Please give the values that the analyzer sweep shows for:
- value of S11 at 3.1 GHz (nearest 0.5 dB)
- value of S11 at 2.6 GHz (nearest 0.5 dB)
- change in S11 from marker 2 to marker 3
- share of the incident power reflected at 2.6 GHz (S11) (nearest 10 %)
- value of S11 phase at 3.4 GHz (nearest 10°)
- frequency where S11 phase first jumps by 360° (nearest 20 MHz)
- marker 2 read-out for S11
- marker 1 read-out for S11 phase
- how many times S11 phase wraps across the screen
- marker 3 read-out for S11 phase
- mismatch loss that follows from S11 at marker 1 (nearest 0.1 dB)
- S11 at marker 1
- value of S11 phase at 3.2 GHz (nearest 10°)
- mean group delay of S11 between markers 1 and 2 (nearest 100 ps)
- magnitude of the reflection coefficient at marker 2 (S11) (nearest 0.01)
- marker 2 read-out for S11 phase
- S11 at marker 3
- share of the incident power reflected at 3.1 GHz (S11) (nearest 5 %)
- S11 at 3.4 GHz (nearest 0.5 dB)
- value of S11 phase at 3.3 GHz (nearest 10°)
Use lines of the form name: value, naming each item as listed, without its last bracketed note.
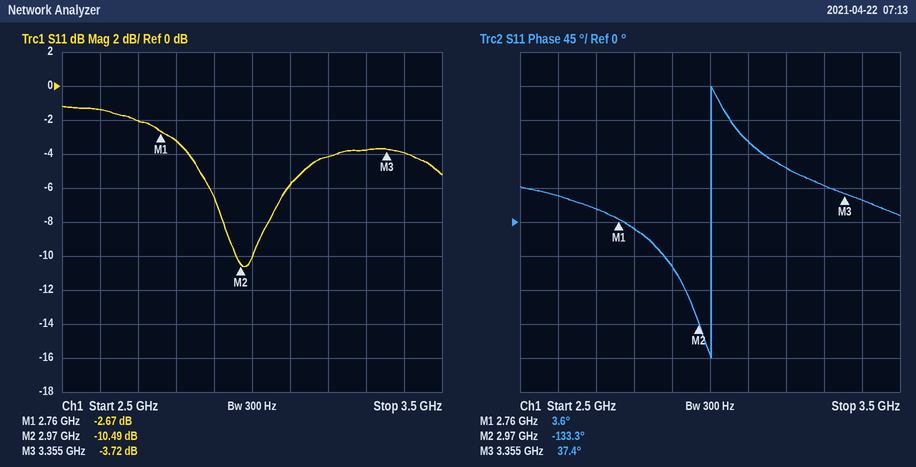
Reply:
value of S11 at 3.1 GHz: -6.0 dB
value of S11 at 2.6 GHz: -1.5 dB
change in S11 from marker 2 to marker 3: 6.77 dB
share of the incident power reflected at 2.6 GHz (S11): 70 %
value of S11 phase at 3.4 GHz: 30°
frequency where S11 phase first jumps by 360°: 3.00 GHz
marker 2 read-out for S11: -10.49 dB
marker 1 read-out for S11 phase: 3.6°
how many times S11 phase wraps across the screen: 1
marker 3 read-out for S11 phase: 37.4°
mismatch loss that follows from S11 at marker 1: 3.4 dB
S11 at marker 1: -2.67 dB
value of S11 phase at 3.2 GHz: 70°
mean group delay of S11 between markers 1 and 2: 1.8 ns
magnitude of the reflection coefficient at marker 2 (S11): 0.30
marker 2 read-out for S11 phase: -133.3°
S11 at marker 3: -3.72 dB
share of the incident power reflected at 3.1 GHz (S11): 25 %
S11 at 3.4 GHz: -4.0 dB
value of S11 phase at 3.3 GHz: 50°
